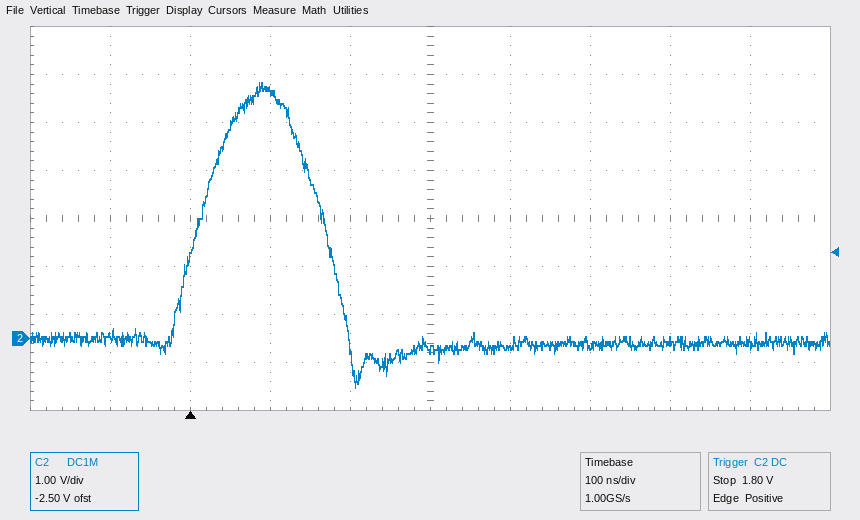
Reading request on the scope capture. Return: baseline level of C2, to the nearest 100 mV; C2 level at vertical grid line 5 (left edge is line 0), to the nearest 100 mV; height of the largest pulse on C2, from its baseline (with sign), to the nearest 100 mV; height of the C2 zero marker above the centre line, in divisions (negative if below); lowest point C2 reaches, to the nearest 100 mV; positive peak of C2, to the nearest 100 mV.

-100 mV
-200 mV
+5.4 V
-2.5 div
-1.0 V
5.3 V
